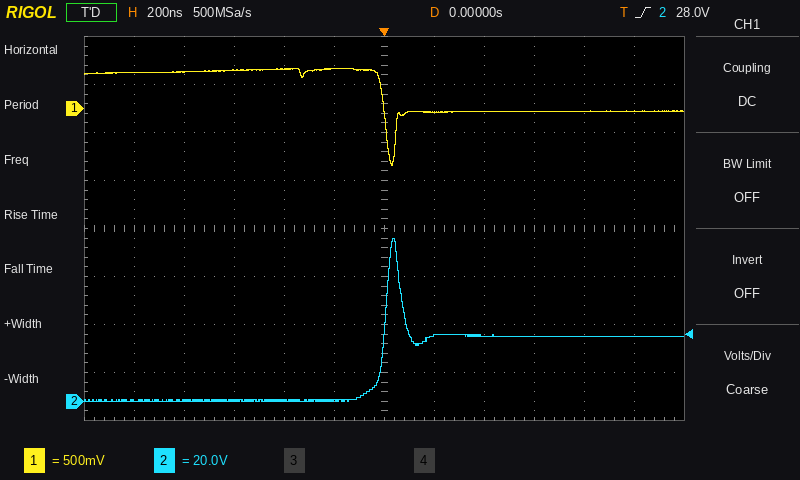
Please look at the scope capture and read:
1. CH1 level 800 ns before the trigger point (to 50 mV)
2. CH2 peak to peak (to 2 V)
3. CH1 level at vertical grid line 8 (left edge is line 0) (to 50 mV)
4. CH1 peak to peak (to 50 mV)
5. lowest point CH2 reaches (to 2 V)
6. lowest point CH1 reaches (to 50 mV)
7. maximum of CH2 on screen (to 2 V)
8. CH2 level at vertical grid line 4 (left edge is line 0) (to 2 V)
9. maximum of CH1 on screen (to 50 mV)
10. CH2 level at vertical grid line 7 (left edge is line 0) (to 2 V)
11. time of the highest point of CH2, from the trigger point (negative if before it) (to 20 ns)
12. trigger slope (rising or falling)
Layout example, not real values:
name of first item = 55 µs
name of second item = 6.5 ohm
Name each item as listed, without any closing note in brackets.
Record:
CH1 level 800 ns before the trigger point = 400 mV
CH2 peak to peak = 68 V
CH1 level at vertical grid line 8 (left edge is line 0) = -50 mV
CH1 peak to peak = 1.00 V
lowest point CH2 reaches = 0 V
lowest point CH1 reaches = -600 mV
maximum of CH2 on screen = 68 V
CH2 level at vertical grid line 4 (left edge is line 0) = 0 V
maximum of CH1 on screen = 400 mV
CH2 level at vertical grid line 7 (left edge is line 0) = 28 V
time of the highest point of CH2, from the trigger point (negative if before it) = +40 ns
trigger slope = rising
